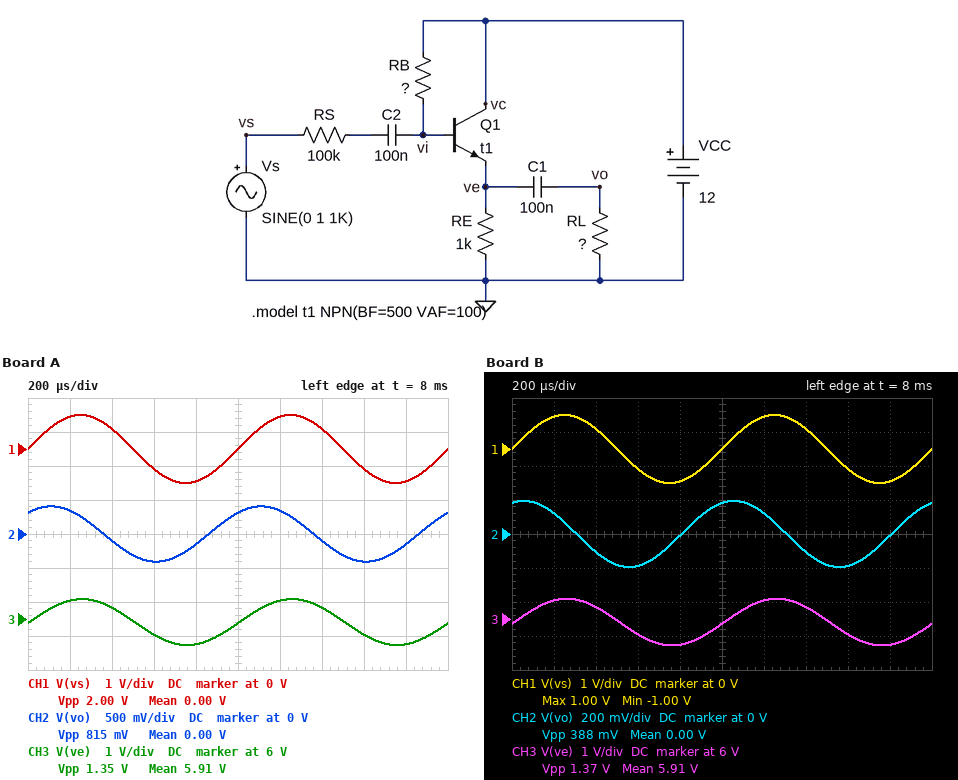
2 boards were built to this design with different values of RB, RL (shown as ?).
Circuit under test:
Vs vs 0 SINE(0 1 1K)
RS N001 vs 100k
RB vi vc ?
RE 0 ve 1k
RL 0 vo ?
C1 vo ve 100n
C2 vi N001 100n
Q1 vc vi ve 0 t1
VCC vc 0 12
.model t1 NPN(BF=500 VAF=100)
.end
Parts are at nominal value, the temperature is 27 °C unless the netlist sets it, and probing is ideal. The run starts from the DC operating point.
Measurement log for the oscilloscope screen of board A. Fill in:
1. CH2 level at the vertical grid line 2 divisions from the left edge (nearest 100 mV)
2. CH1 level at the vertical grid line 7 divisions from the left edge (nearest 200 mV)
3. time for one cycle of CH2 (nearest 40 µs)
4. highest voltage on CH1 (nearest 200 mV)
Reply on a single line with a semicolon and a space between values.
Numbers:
-100 mV; 600 mV; 1.00 ms; 1.0 V
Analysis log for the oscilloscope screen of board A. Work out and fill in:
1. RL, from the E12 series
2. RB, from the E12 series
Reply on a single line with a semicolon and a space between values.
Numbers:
1.2 kΩ; 470 kΩ
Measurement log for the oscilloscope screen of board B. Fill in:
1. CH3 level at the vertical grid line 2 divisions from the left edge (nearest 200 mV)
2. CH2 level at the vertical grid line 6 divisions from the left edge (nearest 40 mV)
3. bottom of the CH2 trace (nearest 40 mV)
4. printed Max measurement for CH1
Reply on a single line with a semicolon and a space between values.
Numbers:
6.4 V; 120 mV; -200 mV; 1.00 V
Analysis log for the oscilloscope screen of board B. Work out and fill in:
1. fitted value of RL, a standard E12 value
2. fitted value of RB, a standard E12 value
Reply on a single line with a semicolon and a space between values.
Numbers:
470 Ω; 470 kΩ
